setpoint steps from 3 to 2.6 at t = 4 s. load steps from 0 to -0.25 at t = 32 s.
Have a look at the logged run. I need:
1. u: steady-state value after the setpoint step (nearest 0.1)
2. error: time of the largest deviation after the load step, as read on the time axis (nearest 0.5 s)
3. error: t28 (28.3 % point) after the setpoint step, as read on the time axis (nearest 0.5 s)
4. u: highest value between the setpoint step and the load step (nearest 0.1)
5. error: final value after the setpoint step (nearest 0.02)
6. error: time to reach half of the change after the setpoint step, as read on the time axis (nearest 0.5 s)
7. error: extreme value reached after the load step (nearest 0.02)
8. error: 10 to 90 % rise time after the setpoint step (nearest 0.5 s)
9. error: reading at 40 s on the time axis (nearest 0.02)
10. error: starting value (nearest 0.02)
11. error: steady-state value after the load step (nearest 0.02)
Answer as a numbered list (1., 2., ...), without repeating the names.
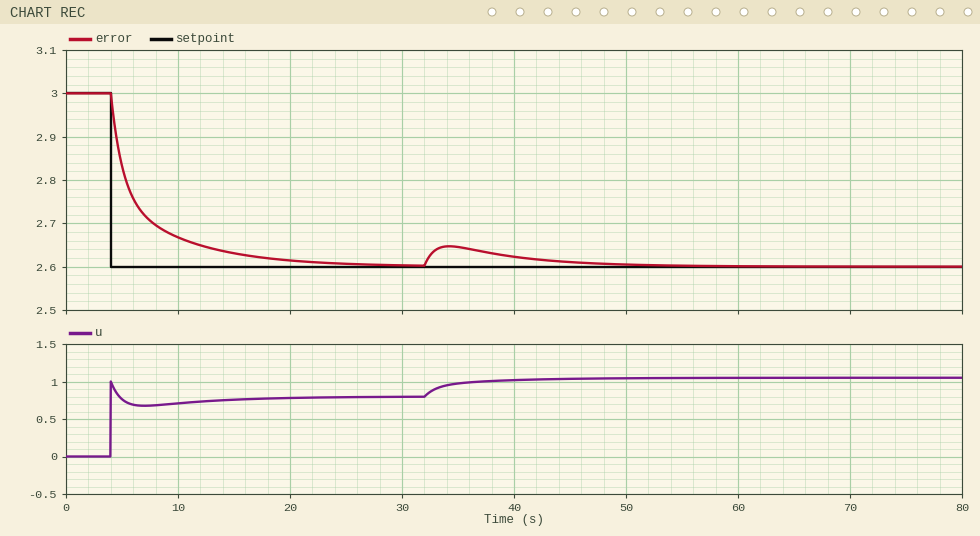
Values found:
1. 0.8
2. 34.0 s
3. 4.5 s
4. 1.0
5. 2.60
6. 5.5 s
7. 2.64
8. 9.0 s
9. 2.62
10. 3.00
11. 2.60
